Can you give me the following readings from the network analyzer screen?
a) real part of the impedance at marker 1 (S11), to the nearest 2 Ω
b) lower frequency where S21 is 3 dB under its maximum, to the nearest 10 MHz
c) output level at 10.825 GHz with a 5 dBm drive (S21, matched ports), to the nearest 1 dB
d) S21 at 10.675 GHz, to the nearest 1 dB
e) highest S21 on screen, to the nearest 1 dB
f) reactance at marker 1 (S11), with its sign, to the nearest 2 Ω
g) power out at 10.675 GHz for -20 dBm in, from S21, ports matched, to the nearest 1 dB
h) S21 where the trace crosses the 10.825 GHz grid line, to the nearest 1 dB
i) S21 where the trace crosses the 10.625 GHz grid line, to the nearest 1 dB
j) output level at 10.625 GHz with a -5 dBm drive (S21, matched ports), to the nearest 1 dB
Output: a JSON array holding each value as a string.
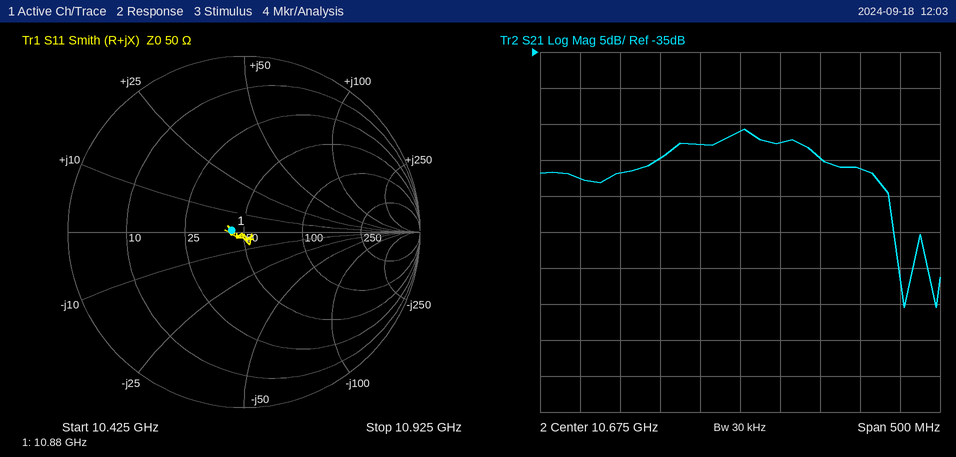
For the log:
["44 Ω", "10.59 GHz", "-46 dBm", "-46 dB", "-46 dB", "0 Ω", "-66 dBm", "-51 dB", "-48 dB", "-53 dBm"]
